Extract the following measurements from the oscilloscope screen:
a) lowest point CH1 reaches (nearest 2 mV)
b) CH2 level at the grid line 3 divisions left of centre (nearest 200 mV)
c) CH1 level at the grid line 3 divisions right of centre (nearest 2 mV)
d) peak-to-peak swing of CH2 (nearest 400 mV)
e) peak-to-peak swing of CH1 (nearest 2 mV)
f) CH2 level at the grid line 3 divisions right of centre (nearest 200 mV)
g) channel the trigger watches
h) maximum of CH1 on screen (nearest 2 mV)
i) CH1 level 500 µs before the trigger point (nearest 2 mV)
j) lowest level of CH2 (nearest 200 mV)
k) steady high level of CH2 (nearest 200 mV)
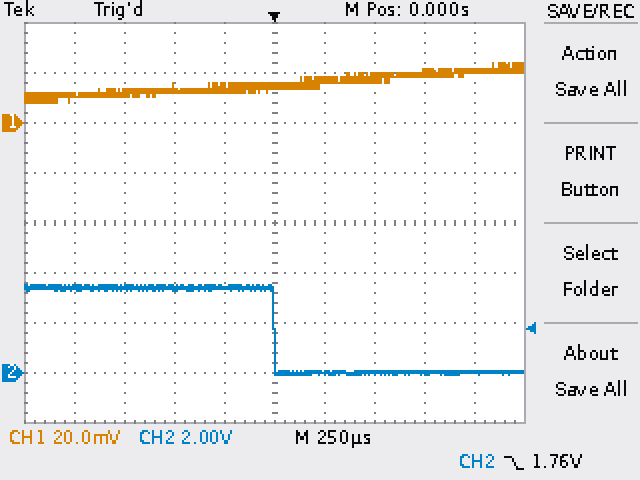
8 mV
3.4 V
20 mV
3.6 V
16 mV
0.0 V
CH2
24 mV
14 mV
0.0 V
3.4 V
